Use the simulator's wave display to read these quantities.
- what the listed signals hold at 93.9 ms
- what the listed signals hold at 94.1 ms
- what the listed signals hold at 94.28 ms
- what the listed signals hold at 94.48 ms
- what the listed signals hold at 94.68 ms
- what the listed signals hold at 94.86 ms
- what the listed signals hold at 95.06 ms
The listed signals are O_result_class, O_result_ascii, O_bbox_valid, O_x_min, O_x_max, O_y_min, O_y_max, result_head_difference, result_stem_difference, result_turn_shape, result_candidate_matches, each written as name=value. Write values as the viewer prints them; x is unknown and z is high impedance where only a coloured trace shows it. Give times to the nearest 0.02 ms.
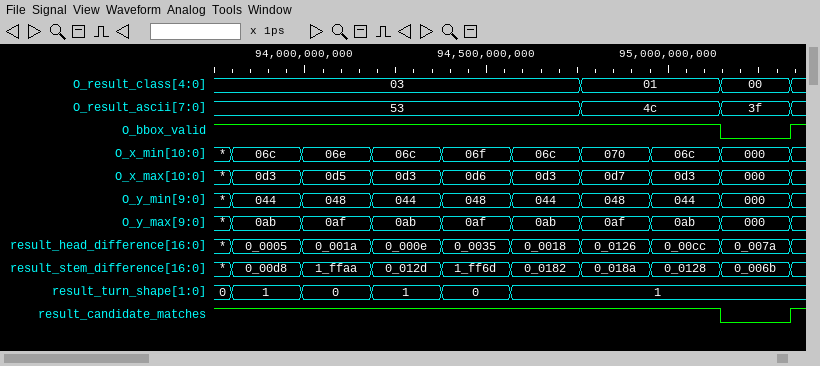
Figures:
O_result_class=03, O_result_ascii=53, O_bbox_valid=1, O_x_min=06c, O_x_max=0d3, O_y_min=044, O_y_max=0ab, result_head_difference=0_0005, result_stem_difference=0_00d8, result_turn_shape=1, result_candidate_matches=1
O_result_class=03, O_result_ascii=53, O_bbox_valid=1, O_x_min=06e, O_x_max=0d5, O_y_min=048, O_y_max=0af, result_head_difference=0_001a, result_stem_difference=1_ffaa, result_turn_shape=0, result_candidate_matches=1
O_result_class=03, O_result_ascii=53, O_bbox_valid=1, O_x_min=06c, O_x_max=0d3, O_y_min=044, O_y_max=0ab, result_head_difference=0_000e, result_stem_difference=0_012d, result_turn_shape=1, result_candidate_matches=1
O_result_class=03, O_result_ascii=53, O_bbox_valid=1, O_x_min=06f, O_x_max=0d6, O_y_min=048, O_y_max=0af, result_head_difference=0_0035, result_stem_difference=1_ff6d, result_turn_shape=0, result_candidate_matches=1
O_result_class=03, O_result_ascii=53, O_bbox_valid=1, O_x_min=06c, O_x_max=0d3, O_y_min=044, O_y_max=0ab, result_head_difference=0_0018, result_stem_difference=0_0182, result_turn_shape=1, result_candidate_matches=1
O_result_class=01, O_result_ascii=4c, O_bbox_valid=1, O_x_min=070, O_x_max=0d7, O_y_min=048, O_y_max=0af, result_head_difference=0_0126, result_stem_difference=0_018a, result_turn_shape=1, result_candidate_matches=1
O_result_class=01, O_result_ascii=4c, O_bbox_valid=1, O_x_min=06c, O_x_max=0d3, O_y_min=044, O_y_max=0ab, result_head_difference=0_00cc, result_stem_difference=0_0128, result_turn_shape=1, result_candidate_matches=1
